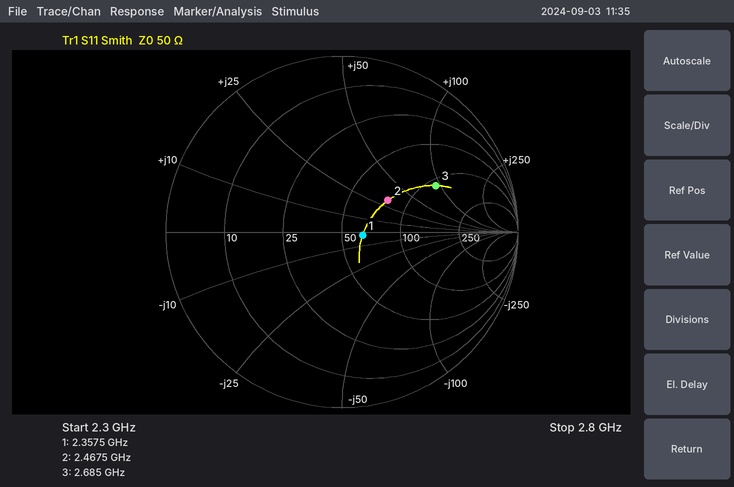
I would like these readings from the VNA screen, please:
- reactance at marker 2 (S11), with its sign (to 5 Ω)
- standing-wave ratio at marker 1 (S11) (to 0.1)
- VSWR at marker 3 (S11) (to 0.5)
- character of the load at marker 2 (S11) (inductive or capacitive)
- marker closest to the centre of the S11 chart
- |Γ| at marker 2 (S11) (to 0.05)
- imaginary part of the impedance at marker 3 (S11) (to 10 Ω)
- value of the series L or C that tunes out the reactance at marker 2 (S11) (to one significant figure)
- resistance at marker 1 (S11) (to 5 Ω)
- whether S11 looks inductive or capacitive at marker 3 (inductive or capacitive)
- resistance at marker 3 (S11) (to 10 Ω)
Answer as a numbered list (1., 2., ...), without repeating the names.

1. +30 Ω
2. 1.3
3. 4.0
4. inductive
5. marker 1
6. 0.30
7. +90 Ω
8. 2 pF
9. 65 Ω
10. inductive
11. 110 Ω
